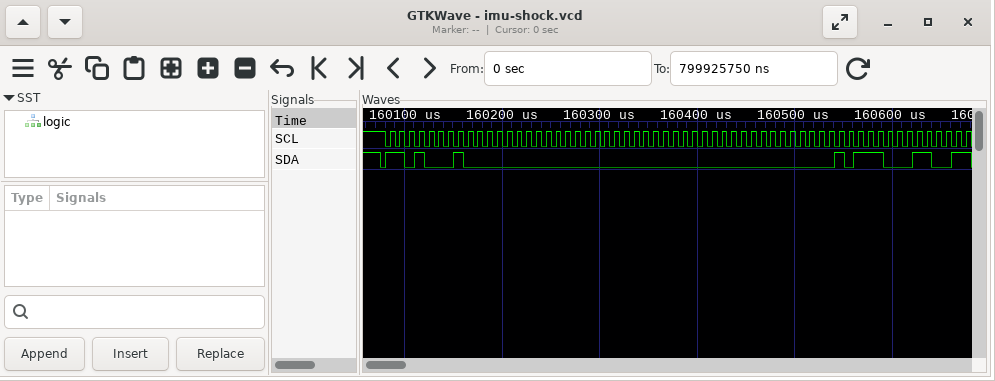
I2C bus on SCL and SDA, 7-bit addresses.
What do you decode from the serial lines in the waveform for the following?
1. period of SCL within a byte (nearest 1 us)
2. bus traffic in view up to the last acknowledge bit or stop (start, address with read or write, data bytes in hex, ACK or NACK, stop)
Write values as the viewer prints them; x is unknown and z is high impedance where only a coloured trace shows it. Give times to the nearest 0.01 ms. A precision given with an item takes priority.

10 us
start, address 68 read ACK, 00 ACK, 00 ACK, 00 ACK, 00 ACK, 5C ACK
